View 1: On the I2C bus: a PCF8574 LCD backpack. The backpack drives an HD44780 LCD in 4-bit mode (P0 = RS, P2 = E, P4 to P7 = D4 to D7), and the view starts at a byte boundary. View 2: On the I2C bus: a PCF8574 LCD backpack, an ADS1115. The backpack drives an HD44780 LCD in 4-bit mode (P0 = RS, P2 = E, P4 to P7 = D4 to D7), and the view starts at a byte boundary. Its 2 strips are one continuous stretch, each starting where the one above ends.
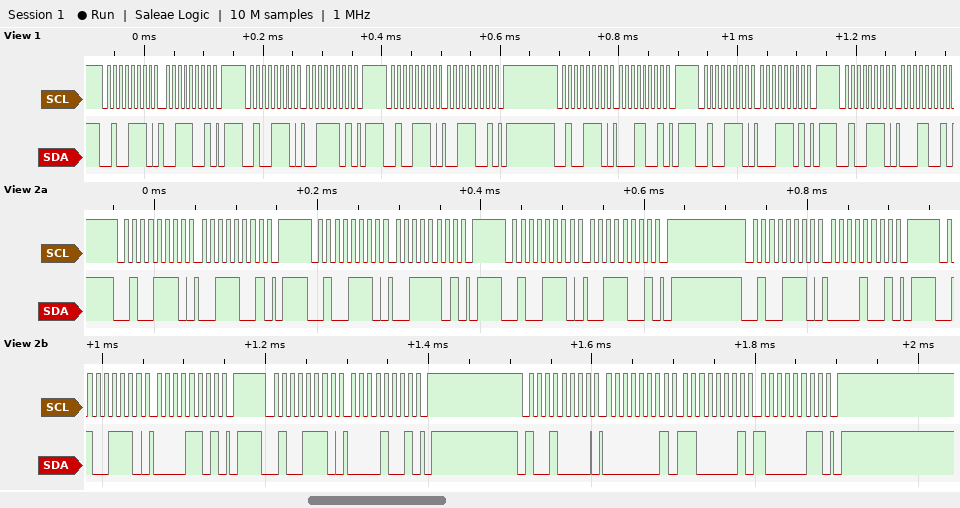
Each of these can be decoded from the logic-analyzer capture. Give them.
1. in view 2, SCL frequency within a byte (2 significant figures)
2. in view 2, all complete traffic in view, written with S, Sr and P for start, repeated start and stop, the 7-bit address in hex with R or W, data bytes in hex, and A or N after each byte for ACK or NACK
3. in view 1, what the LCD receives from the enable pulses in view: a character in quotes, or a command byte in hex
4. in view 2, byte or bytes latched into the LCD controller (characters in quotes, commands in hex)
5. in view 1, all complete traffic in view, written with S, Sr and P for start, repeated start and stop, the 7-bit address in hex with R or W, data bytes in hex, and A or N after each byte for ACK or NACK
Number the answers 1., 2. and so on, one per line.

1. 100 kHz
2. S 27W A 39 A P S 27W A 3D A P S 27W A 39 A P S 27W A 09 A P S 27W A 0D A P S 27W A 09 A P S 48W A 01 A C1 A 83 A P
3. '1'
4. '0'
5. S 27W A 39 A P S 27W A 3D A P S 27W A 39 A P S 27W A 19 A P S 27W A 1D A P S 27W A 19 A
